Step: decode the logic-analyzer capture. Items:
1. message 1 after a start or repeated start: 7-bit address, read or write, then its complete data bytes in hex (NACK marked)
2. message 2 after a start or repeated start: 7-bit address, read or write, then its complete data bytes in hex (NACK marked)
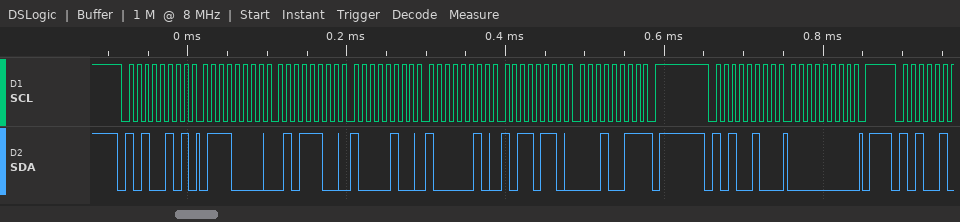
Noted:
0x52 read: 70 5C 84 82 B6 13 NACK
0x52 write: 00
